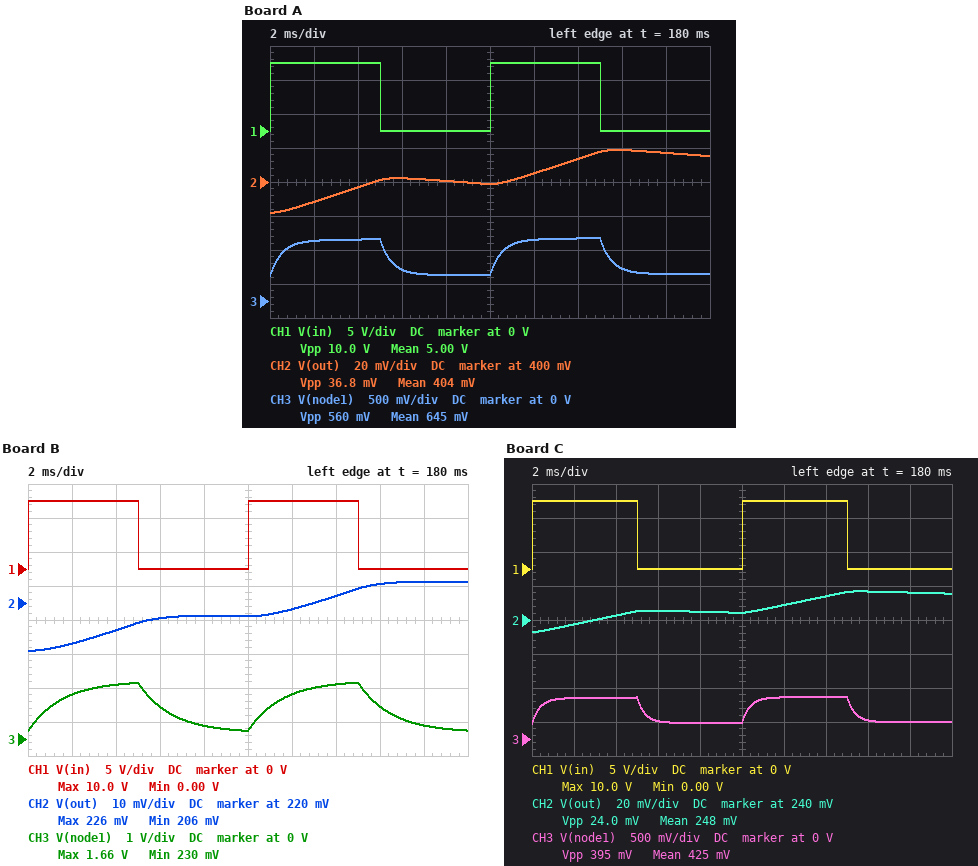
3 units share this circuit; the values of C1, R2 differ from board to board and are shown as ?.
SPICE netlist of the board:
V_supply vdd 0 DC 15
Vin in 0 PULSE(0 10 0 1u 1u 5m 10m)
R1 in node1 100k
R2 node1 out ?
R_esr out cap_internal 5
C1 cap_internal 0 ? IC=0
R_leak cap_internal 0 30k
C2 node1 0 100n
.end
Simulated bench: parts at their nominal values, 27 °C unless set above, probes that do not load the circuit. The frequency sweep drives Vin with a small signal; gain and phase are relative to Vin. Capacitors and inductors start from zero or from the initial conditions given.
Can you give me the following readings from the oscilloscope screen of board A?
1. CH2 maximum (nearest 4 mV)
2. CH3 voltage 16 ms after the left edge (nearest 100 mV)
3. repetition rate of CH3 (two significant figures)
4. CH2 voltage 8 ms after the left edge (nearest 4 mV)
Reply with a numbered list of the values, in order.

1. 420 mV
2. 500 mV
3. 100 Hz
4. 400 mV
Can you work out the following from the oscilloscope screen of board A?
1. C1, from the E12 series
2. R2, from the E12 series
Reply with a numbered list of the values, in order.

1. 18 µF
2. 5.6 kΩ
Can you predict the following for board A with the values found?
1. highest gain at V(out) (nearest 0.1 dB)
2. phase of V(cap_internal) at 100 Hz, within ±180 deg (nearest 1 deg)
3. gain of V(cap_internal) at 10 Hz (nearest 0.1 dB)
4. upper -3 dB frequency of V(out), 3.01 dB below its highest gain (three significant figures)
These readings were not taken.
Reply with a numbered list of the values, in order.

1. -13.1 dB
2. -108 deg
3. -41.6 dB
4. 377 mHz
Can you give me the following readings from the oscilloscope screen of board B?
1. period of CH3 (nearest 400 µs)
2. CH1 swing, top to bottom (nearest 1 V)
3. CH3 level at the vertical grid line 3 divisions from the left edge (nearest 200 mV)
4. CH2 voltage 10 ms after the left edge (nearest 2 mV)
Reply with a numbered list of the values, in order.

1. 10.0 ms
2. 10 V
3. 1.0 V
4. 216 mV
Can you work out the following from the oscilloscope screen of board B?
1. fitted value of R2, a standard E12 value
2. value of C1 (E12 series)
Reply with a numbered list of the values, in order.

1. 18 kΩ
2. 33 µF
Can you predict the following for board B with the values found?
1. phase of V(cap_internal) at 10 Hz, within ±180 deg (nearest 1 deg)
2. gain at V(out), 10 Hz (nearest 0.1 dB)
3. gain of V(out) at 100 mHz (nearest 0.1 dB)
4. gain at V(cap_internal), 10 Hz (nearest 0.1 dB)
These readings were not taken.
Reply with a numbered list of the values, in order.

1. -94 deg
2. -47.8 dB
3. -14.8 dB
4. -47.8 dB
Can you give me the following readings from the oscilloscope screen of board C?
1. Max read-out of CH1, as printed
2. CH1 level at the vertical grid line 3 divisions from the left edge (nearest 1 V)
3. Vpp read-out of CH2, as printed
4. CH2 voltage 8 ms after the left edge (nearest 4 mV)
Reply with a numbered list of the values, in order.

1. 10.0 V
2. 0 V
3. 24.0 mV
4. 244 mV
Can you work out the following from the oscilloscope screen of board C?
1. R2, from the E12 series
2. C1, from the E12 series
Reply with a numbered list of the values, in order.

1. 3.9 kΩ
2. 33 µF
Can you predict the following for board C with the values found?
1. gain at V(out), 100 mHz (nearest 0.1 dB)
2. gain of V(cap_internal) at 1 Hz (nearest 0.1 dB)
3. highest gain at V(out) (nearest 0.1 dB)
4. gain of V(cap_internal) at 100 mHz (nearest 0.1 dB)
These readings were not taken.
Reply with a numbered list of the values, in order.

1. -13.9 dB
2. -26.9 dB
3. -13.0 dB
4. -13.9 dB
